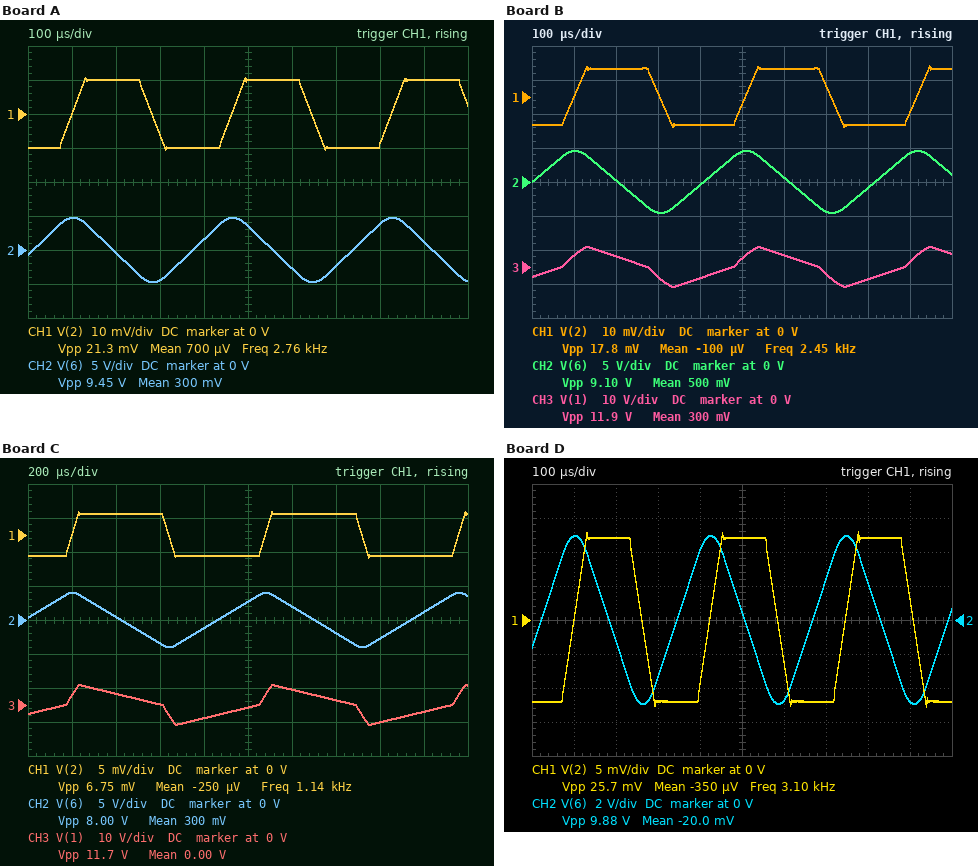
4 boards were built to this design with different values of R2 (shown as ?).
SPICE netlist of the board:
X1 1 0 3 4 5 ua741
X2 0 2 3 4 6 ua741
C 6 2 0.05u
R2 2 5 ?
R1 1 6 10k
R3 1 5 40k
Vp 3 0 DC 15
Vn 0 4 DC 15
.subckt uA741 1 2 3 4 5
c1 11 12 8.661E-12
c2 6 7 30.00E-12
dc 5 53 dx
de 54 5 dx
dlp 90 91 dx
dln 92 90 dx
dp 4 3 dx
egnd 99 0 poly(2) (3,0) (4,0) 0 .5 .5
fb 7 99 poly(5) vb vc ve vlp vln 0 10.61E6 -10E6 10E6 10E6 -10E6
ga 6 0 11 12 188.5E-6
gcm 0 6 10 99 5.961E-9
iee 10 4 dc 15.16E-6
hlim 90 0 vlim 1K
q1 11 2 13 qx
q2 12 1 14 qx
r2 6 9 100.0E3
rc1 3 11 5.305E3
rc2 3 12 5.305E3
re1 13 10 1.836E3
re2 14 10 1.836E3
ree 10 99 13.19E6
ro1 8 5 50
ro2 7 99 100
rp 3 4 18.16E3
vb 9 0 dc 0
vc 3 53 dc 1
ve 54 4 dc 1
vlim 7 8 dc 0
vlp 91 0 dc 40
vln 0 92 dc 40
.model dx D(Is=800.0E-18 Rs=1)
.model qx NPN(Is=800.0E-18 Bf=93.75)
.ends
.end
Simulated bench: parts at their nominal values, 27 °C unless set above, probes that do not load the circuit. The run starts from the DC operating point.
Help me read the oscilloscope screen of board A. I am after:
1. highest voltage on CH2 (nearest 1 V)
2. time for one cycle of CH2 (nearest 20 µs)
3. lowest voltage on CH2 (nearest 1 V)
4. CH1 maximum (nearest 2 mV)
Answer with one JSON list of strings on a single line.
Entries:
["5 V", "360 µs", "-5 V", "10 mV"]
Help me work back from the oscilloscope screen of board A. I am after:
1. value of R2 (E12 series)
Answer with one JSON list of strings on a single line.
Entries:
["4.7 kΩ"]
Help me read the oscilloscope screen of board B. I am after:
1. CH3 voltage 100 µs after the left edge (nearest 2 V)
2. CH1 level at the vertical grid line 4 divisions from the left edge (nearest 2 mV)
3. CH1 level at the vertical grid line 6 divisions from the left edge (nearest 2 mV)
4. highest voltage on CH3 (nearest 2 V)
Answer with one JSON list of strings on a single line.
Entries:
["4 V", "-8 mV", "8 mV", "6 V"]
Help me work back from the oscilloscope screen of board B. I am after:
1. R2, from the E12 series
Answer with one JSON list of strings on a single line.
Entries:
["5.6 kΩ"]
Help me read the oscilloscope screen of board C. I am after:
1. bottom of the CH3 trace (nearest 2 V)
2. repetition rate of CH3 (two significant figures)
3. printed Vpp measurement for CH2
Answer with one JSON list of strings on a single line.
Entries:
["-6 V", "1.1 kHz", "8.00 V"]
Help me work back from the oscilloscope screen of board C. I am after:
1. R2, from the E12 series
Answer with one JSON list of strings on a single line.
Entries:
["15 kΩ"]
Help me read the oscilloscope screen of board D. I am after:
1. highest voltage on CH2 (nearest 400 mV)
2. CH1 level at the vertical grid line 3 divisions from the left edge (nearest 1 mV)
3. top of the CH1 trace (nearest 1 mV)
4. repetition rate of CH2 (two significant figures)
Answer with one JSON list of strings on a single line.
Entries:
["4.8 V", "-12 mV", "13 mV", "3.1 kHz"]
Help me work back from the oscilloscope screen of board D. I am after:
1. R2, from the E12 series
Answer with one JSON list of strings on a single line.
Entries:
["3.9 kΩ"]
